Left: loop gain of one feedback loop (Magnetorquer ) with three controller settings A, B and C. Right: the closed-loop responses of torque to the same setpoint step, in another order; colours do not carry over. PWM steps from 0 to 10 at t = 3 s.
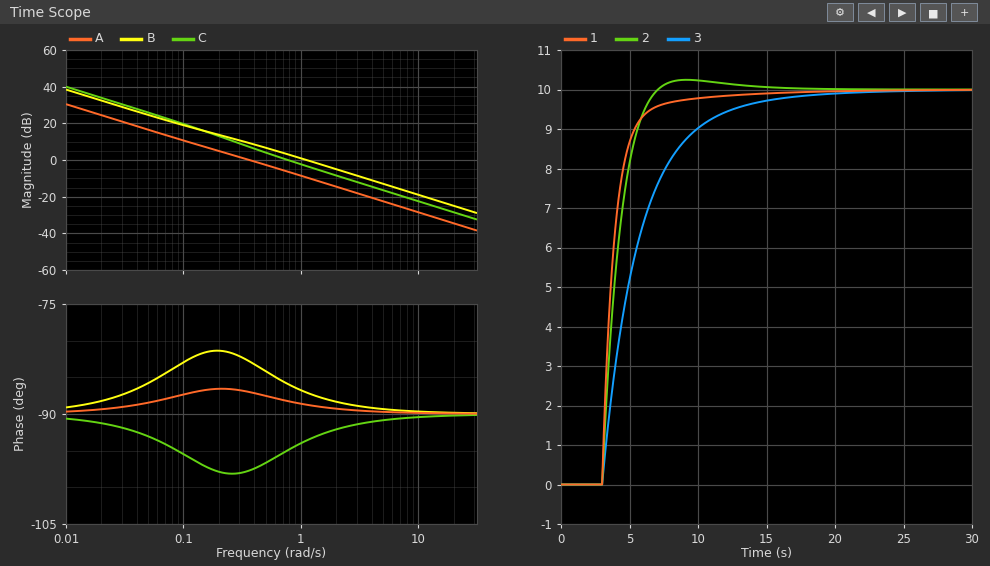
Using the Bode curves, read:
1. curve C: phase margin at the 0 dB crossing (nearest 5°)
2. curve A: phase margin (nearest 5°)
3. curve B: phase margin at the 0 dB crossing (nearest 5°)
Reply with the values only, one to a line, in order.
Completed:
85°
95°
95°
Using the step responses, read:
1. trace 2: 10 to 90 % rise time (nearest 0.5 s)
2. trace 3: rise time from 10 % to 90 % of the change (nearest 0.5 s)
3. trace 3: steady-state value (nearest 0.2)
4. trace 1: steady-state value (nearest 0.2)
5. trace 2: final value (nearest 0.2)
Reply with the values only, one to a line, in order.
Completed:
2.5 s
6.5 s
10.0
10.0
10.0
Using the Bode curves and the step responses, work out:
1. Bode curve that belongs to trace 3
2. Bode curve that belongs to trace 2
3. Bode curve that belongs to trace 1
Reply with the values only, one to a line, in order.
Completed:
A
C
B
